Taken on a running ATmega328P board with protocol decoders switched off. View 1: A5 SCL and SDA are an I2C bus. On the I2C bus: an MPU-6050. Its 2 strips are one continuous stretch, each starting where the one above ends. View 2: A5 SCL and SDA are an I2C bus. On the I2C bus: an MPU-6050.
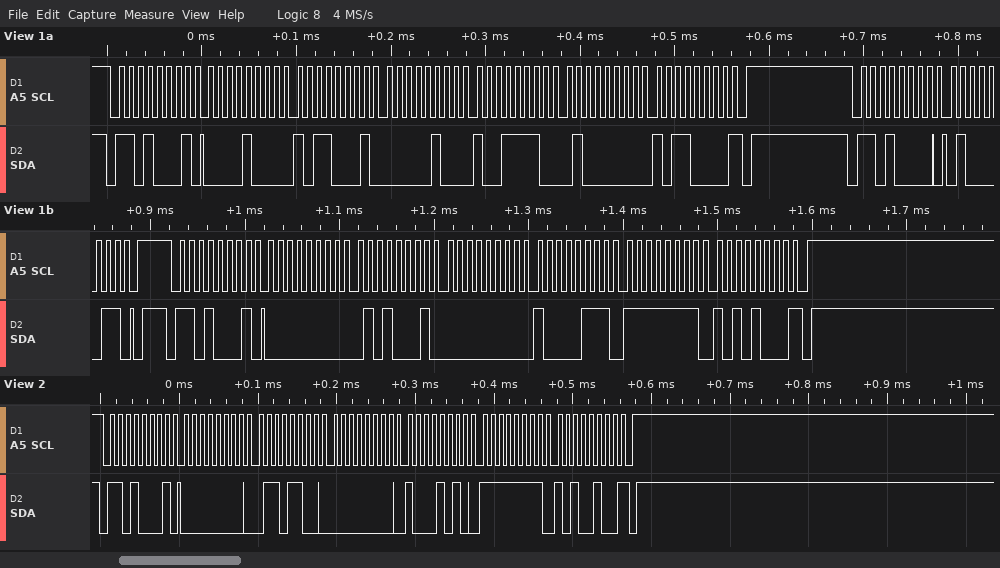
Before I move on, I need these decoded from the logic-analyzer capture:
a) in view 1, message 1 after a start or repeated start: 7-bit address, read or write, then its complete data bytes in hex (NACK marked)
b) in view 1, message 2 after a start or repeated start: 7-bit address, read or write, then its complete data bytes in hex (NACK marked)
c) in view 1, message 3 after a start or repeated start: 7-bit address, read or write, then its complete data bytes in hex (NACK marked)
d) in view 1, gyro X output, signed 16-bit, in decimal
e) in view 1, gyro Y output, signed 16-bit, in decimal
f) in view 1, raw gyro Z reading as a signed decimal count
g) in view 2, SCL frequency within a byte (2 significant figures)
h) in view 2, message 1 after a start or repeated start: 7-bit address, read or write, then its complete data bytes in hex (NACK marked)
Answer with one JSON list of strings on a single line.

["0x68 read: 08 B1 04 9E 40 B0 NACK", "0x68 write: 43", "0x68 read: 00 51 00 87 FF A8 NACK", "81", "135", "-88", "100 kHz", "0x68 read: 00 6C 00 8A FF A4 NACK"]
